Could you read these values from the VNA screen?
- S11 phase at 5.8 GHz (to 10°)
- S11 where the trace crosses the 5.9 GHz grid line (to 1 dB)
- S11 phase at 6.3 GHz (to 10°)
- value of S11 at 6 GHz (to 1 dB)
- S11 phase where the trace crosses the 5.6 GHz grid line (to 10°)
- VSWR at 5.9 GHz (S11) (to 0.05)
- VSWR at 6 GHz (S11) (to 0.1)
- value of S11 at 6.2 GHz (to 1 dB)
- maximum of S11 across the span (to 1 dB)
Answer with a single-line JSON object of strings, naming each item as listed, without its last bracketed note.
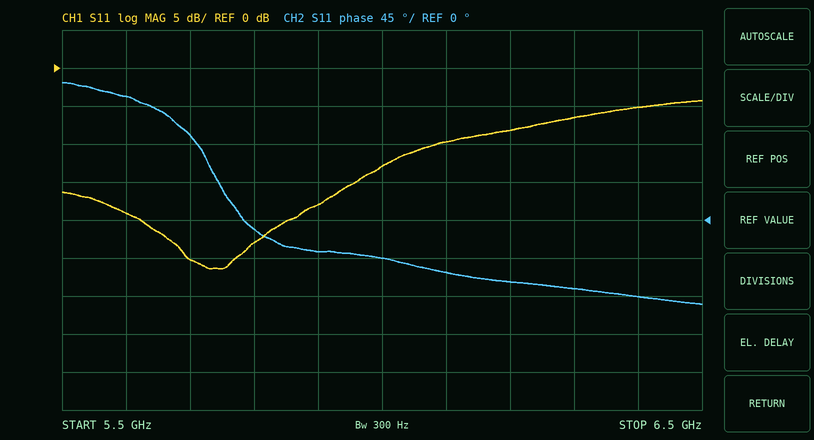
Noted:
{"S11 phase at 5.8 GHz": "-10°", "S11 where the trace crosses the 5.9 GHz grid line": "-18 dB", "S11 phase at 6.3 GHz": "-80°", "value of S11 at 6 GHz": "-13 dB", "S11 phase where the trace crosses the 5.6 GHz grid line": "150°", "VSWR at 5.9 GHz (S11)": "1.30", "VSWR at 6 GHz (S11)": "1.6", "value of S11 at 6.2 GHz": "-8 dB", "maximum of S11 across the span": "-4 dB"}
